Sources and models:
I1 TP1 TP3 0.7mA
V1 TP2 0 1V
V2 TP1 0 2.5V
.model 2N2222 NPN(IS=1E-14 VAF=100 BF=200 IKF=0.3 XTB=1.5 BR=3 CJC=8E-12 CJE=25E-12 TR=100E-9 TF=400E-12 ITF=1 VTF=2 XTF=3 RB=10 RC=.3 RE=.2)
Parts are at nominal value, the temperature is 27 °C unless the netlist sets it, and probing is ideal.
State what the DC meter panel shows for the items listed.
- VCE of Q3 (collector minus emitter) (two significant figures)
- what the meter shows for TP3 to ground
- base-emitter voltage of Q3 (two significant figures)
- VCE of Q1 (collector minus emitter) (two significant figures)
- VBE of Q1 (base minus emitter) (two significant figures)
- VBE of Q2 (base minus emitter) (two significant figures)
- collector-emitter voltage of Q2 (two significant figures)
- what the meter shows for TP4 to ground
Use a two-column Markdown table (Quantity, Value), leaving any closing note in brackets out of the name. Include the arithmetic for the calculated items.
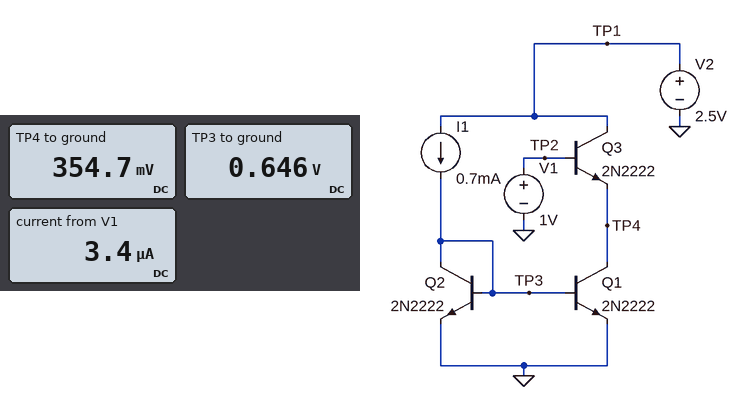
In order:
| Quantity | Value |
|---|---|
| VCE of Q3 (collector minus emitter) | 2.5 V - 354.7 mV = 2.1 V |
| what the meter shows for TP3 to ground | 0.646 V |
| base-emitter voltage of Q3 | 1 V - 354.7 mV = 650 mV |
| VCE of Q1 (collector minus emitter) | 354.7 mV = 350 mV |
| VBE of Q1 (base minus emitter) | 646 mV = 650 mV |
| VBE of Q2 (base minus emitter) | 646 mV = 650 mV |
| collector-emitter voltage of Q2 | 646 mV = 650 mV |
| what the meter shows for TP4 to ground | 354.7 mV |
